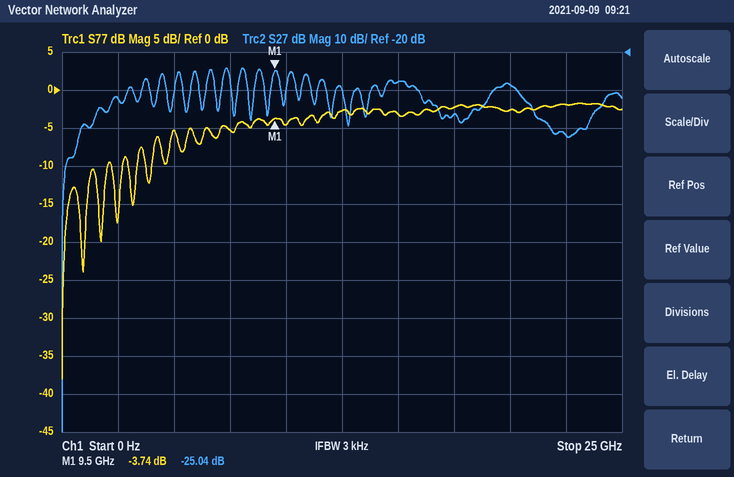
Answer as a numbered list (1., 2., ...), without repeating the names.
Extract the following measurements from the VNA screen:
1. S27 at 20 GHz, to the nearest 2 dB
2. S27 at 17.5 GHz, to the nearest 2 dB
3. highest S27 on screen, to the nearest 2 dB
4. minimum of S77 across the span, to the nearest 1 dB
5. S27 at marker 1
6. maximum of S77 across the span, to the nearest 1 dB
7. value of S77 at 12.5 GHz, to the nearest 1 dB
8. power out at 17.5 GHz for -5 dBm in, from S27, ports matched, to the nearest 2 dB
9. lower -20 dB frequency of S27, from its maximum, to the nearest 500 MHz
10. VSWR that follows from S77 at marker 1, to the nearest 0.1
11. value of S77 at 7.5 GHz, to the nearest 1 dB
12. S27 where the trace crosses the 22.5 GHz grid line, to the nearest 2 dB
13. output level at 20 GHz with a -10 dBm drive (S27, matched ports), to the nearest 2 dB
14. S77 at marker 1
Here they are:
1. -28 dB
2. -36 dB
3. -24 dB
4. -38 dB
5. -25.04 dB
6. -2 dB
7. -3 dB
8. -42 dBm
9. 500 MHz
10. 4.7
11. -5 dB
12. -42 dB
13. -38 dBm
14. -3.74 dB
